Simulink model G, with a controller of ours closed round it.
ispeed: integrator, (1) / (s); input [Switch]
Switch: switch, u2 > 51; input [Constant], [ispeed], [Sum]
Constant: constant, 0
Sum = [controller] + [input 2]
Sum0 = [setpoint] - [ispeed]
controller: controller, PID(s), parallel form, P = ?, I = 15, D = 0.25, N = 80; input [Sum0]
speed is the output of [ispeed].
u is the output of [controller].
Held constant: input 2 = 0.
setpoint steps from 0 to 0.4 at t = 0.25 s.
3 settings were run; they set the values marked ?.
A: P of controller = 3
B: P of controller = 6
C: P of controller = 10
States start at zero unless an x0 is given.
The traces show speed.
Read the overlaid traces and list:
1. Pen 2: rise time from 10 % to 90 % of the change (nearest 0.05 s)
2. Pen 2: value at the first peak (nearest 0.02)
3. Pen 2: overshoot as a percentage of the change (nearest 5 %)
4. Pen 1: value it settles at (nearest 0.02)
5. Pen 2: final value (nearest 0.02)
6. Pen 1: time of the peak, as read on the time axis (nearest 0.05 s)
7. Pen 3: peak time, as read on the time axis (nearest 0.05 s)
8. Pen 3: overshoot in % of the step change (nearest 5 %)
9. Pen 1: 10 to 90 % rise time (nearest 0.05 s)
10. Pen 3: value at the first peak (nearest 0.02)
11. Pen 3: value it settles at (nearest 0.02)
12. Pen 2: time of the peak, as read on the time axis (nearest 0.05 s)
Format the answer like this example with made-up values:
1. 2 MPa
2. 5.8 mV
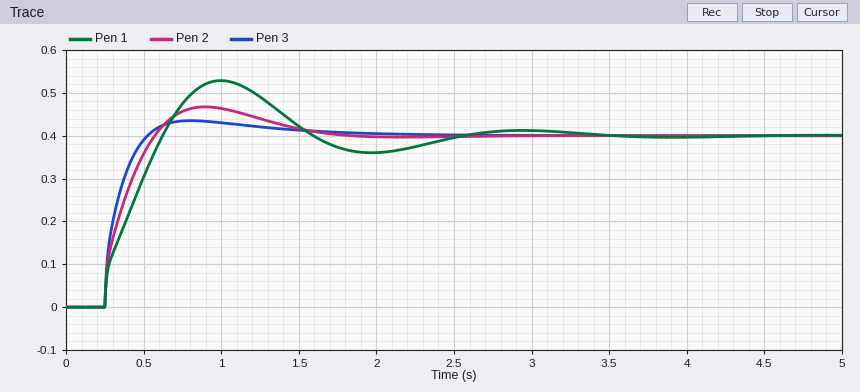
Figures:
1. 0.25 s
2. 0.46
3. 15 %
4. 0.40
5. 0.40
6. 1.00 s
7. 0.80 s
8. 10 %
9. 0.30 s
10. 0.44
11. 0.40
12. 0.90 s
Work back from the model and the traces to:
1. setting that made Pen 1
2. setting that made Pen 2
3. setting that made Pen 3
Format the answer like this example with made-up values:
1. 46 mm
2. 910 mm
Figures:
1. A
2. B
3. C
